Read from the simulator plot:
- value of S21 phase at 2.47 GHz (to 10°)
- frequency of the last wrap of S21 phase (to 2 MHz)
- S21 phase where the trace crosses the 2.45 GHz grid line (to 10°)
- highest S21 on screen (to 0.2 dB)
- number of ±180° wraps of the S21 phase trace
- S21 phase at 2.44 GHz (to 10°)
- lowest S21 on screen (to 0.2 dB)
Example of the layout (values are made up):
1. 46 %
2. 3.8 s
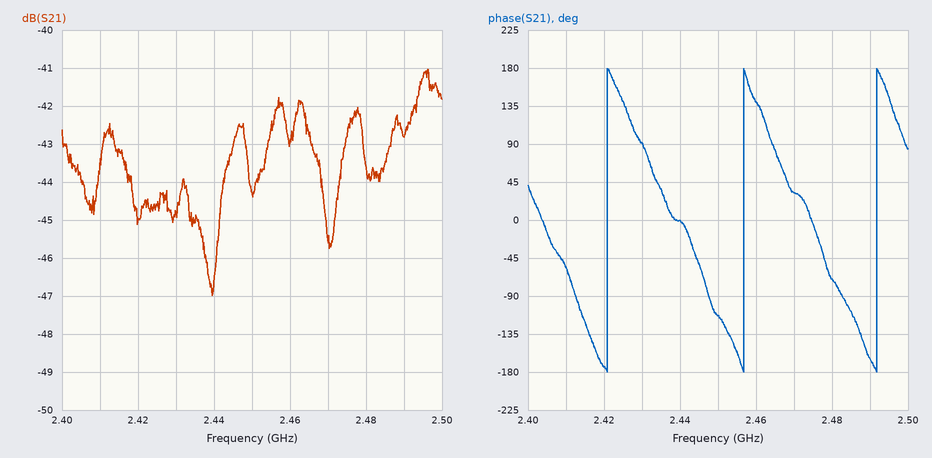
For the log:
1. 30°
2. 2.492 GHz
3. -110°
4. -41.0 dB
5. 3
6. 0°
7. -47.0 dB
